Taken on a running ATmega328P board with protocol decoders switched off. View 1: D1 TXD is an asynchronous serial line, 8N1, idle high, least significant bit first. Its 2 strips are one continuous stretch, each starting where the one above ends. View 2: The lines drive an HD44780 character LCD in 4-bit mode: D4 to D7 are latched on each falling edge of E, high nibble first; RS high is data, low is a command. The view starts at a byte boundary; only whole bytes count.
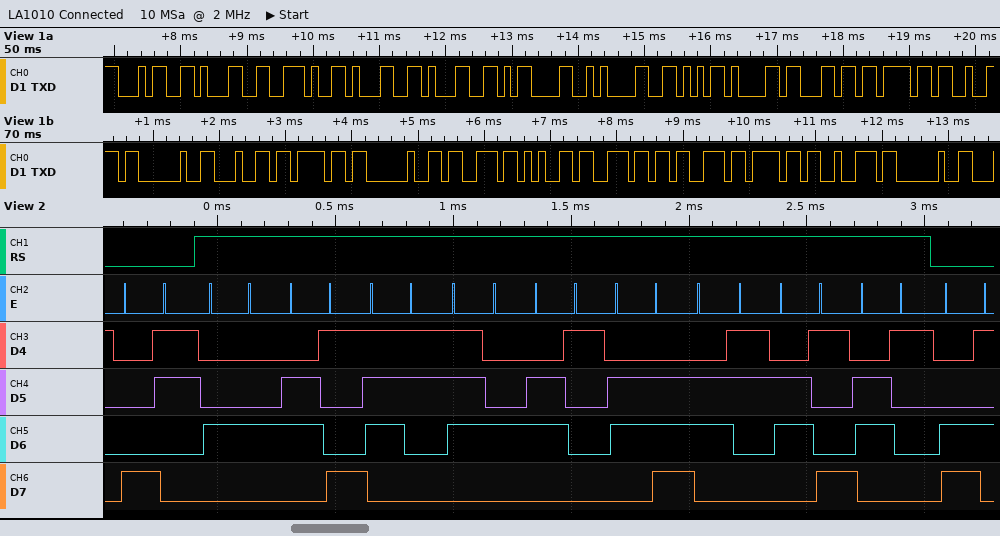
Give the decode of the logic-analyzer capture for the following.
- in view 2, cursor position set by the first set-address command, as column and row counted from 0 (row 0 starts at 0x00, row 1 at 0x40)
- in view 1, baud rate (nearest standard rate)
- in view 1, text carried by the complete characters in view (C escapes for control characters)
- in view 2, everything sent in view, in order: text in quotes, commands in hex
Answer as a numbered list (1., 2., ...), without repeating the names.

1. column 3, row 0
2. 9600 baud
3. "41.11\r\nValor do sensor "
4. 0x83 "Distancia" 0xC5
